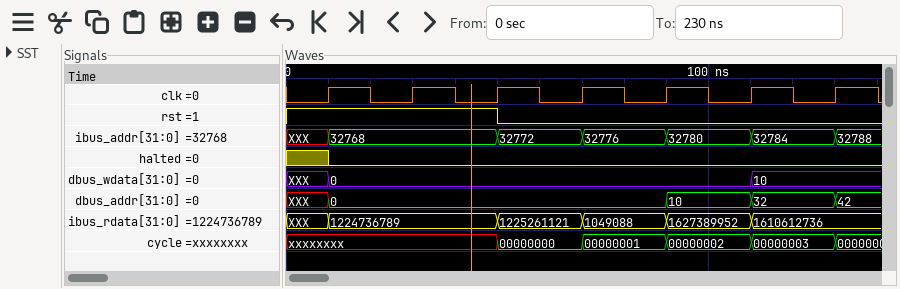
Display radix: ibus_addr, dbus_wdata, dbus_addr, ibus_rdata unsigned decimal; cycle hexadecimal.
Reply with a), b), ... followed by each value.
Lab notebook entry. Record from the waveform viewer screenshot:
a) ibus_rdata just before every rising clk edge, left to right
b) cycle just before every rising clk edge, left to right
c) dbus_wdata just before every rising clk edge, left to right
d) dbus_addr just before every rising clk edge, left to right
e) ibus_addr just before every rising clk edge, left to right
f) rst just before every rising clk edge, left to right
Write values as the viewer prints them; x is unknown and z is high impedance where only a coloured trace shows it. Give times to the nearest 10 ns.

a) XXX, 1224736789, 1224736789, 1225261121, 1049088, 1627389952, 1610612736
b) xxxxxxxx, xxxxxxxx, xxxxxxxx, 00000000, 00000001, 00000002, 00000003
c) XXX, 0, 0, 0, 0, 0, 10
d) XXX, 0, 0, 0, 0, 10, 32
e) XXX, 32768, 32768, 32772, 32776, 32780, 32784
f) 1 1 1 0 0 0 0
